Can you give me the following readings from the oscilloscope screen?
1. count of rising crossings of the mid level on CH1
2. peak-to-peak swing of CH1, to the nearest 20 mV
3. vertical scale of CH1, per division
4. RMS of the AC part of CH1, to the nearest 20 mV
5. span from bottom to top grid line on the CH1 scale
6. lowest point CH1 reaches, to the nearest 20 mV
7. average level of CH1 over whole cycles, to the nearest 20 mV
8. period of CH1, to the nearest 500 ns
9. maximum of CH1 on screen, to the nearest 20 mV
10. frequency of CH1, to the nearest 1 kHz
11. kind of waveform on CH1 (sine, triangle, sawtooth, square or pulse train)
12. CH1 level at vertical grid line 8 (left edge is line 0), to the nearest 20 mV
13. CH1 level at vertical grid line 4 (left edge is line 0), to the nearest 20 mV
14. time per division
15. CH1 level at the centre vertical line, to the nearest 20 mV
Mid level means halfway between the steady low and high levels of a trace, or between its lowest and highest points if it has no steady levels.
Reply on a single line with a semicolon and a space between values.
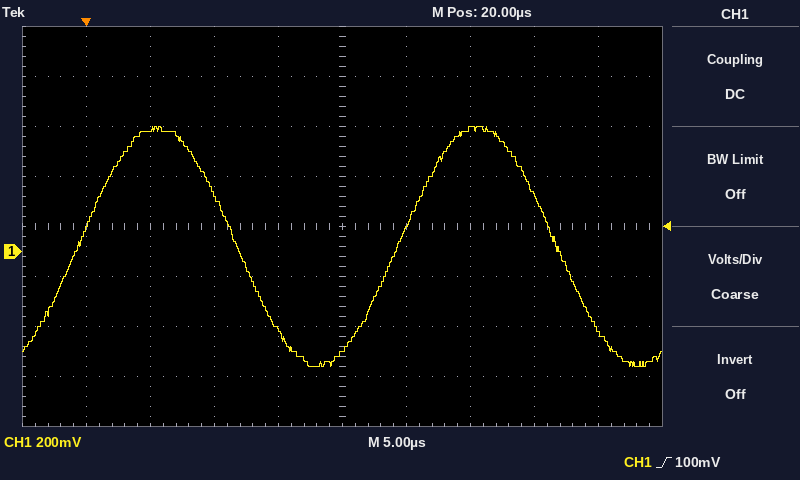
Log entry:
2; 960 mV; 200 mV; 340 mV; 1.6 V; -460 mV; 20 mV; 25.0 µs; 500 mV; 40 kHz; sine; 220 mV; -320 mV; 5 µs; -400 mV
